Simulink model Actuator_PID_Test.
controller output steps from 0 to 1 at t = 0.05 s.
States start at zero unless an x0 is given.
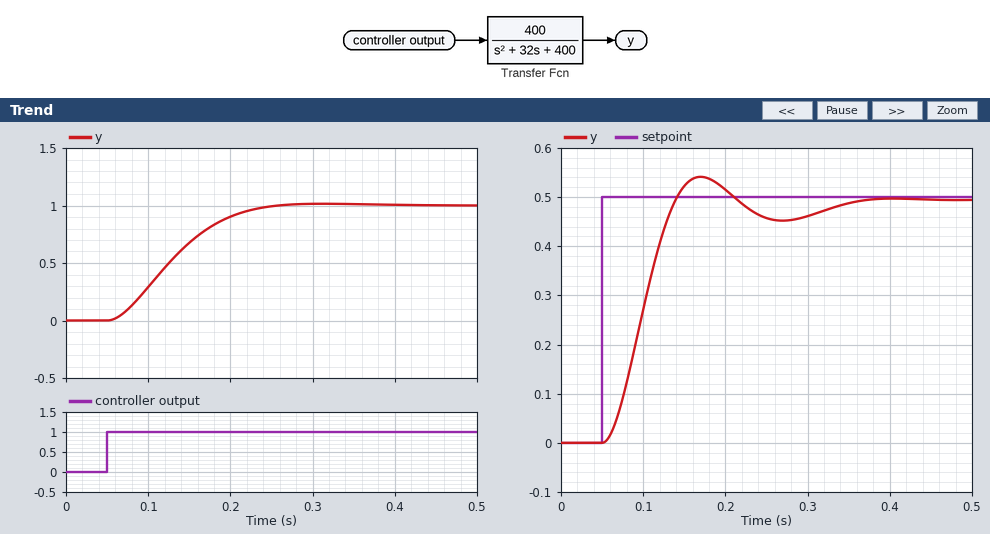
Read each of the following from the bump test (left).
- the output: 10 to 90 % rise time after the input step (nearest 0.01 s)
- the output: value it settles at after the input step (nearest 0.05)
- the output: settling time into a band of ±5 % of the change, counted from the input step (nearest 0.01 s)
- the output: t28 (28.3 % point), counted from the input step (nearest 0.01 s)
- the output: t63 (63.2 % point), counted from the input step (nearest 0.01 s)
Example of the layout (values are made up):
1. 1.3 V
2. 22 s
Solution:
1. 0.12 s
2. 1.00
3. 0.17 s
4. 0.05 s
5. 0.09 s
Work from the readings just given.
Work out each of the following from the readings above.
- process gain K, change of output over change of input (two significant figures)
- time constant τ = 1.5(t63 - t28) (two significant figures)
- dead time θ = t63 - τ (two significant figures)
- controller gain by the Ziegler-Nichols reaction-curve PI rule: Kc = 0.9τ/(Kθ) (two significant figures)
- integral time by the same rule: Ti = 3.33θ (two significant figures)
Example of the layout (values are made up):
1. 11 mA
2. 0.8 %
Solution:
1. 1.0
2. 0.060 s
3. 0.030 s
4. 1.8
5. 0.100 s
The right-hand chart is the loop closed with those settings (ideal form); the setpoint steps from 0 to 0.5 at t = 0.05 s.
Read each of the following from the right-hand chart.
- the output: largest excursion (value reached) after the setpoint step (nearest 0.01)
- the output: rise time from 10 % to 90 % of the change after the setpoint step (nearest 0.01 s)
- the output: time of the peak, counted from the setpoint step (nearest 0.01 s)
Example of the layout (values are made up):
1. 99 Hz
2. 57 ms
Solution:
1. 0.54
2. 0.06 s
3. 0.12 s
